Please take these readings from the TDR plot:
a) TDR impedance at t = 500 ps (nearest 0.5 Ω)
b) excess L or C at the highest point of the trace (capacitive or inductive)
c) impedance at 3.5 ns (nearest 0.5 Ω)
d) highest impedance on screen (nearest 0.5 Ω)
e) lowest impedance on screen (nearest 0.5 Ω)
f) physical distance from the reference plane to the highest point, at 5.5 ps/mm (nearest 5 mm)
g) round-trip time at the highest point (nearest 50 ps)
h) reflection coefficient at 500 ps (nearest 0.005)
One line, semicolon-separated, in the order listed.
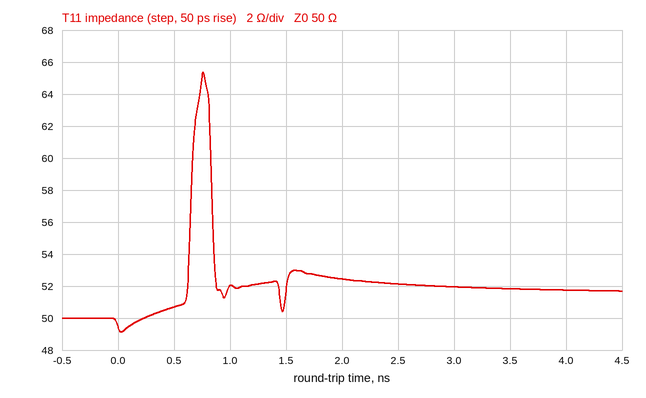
50.5 Ω; inductive; 52.0 Ω; 65.5 Ω; 49.0 Ω; 70 mm; 750 ps; +0.005
